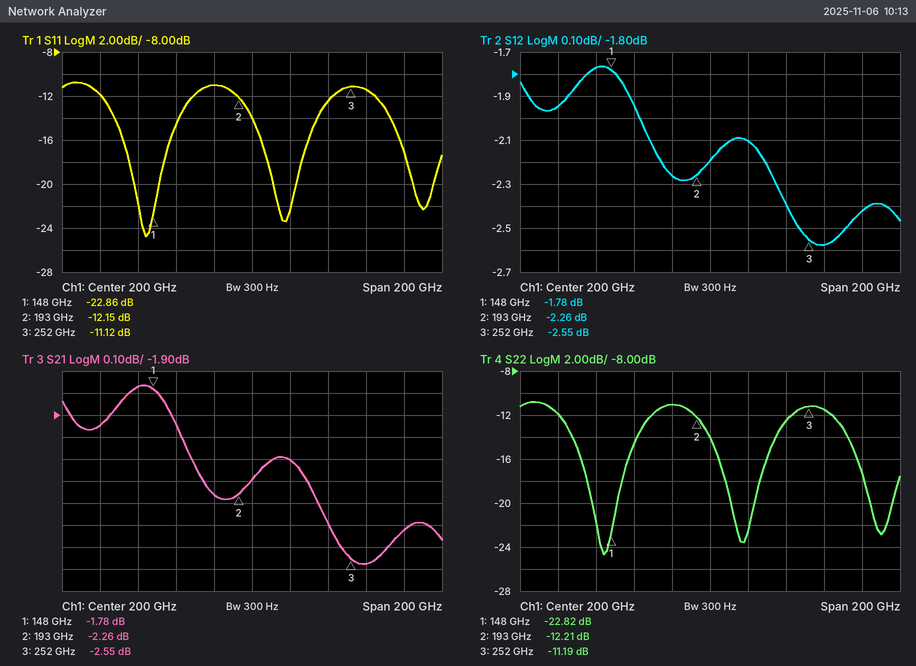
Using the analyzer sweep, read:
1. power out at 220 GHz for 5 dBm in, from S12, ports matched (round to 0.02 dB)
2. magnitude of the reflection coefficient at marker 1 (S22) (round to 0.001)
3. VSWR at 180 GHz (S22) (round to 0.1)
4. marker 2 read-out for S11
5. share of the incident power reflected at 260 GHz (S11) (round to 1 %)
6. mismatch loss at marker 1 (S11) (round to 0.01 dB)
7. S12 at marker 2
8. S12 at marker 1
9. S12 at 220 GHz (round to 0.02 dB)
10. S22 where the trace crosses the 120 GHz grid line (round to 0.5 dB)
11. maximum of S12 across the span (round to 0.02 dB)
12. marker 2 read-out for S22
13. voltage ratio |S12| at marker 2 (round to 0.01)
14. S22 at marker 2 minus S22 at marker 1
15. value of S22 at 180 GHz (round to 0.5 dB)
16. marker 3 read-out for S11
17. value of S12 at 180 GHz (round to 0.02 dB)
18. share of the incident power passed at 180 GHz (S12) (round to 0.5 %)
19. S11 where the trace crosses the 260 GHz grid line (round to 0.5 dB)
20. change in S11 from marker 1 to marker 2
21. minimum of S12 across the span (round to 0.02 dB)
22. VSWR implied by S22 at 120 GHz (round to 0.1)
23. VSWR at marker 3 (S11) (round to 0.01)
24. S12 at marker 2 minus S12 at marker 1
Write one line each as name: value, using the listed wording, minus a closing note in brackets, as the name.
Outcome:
power out at 220 GHz for 5 dBm in, from S12, ports matched: 2.90 dBm
magnitude of the reflection coefficient at marker 1 (S22): 0.072
VSWR at 180 GHz (S22): 1.8
marker 2 read-out for S11: -12.15 dB
share of the incident power reflected at 260 GHz (S11): 7 %
mismatch loss at marker 1 (S11): 0.02 dB
S12 at marker 2: -2.26 dB
S12 at marker 1: -1.78 dB
S12 at 220 GHz: -2.10 dB
S22 where the trace crosses the 120 GHz grid line: -12.0 dB
maximum of S12 across the span: -1.76 dB
marker 2 read-out for S22: -12.21 dB
voltage ratio |S12| at marker 2: 0.77
S22 at marker 2 minus S22 at marker 1: 10.61 dB
value of S22 at 180 GHz: -11.0 dB
marker 3 read-out for S11: -11.12 dB
value of S12 at 180 GHz: -2.26 dB
share of the incident power passed at 180 GHz (S12): 59.5 %
S11 where the trace crosses the 260 GHz grid line: -11.5 dB
change in S11 from marker 1 to marker 2: 10.71 dB
minimum of S12 across the span: -2.58 dB
VSWR implied by S22 at 120 GHz: 1.7
VSWR at marker 3 (S11): 1.77
S12 at marker 2 minus S12 at marker 1: -0.48 dB
